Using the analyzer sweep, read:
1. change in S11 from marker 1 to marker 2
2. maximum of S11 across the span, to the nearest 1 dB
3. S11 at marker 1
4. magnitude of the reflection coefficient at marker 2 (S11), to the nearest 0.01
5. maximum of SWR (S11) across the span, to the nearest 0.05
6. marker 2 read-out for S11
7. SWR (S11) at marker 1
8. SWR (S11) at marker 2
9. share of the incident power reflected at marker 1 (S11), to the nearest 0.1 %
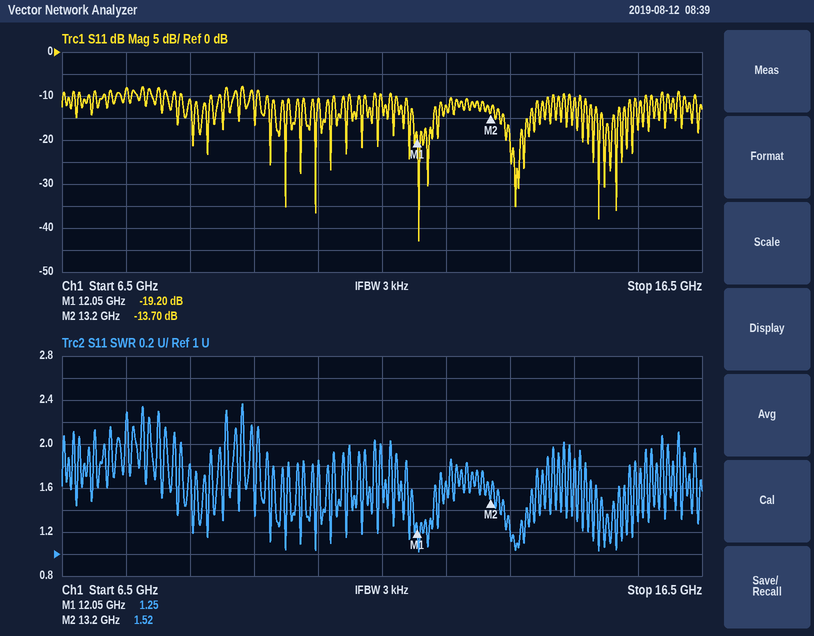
5.50 dB
-8 dB
-19.20 dB
0.21
2.35
-13.70 dB
1.25
1.52
1.2 %
